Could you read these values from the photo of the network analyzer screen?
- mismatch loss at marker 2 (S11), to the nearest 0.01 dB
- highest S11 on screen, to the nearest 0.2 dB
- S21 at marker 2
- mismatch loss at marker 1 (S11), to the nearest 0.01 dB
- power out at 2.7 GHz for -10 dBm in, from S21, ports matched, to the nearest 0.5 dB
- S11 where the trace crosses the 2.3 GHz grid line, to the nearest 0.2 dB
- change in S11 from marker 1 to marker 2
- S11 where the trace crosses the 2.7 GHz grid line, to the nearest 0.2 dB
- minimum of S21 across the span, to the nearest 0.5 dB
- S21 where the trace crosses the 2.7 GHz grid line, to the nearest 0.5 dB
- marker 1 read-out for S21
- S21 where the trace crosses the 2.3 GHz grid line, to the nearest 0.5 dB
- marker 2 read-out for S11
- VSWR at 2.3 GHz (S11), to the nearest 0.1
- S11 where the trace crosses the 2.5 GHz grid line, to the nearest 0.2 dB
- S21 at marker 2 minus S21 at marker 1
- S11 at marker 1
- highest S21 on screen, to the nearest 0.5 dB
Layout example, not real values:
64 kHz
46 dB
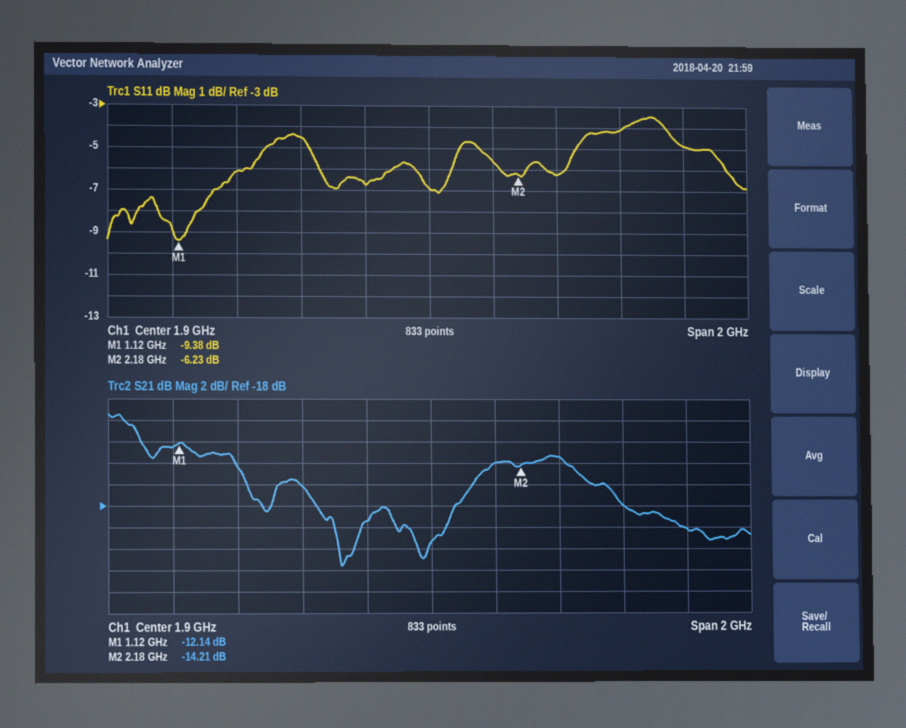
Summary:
1.18 dB
-3.4 dB
-14.21 dB
0.53 dB
-30.0 dBm
-6.2 dB
3.15 dB
-4.8 dB
-23.5 dB
-20.0 dB
-12.14 dB
-13.5 dB
-6.23 dB
2.9
-4.2 dB
-2.07 dB
-9.38 dB
-9.5 dB
